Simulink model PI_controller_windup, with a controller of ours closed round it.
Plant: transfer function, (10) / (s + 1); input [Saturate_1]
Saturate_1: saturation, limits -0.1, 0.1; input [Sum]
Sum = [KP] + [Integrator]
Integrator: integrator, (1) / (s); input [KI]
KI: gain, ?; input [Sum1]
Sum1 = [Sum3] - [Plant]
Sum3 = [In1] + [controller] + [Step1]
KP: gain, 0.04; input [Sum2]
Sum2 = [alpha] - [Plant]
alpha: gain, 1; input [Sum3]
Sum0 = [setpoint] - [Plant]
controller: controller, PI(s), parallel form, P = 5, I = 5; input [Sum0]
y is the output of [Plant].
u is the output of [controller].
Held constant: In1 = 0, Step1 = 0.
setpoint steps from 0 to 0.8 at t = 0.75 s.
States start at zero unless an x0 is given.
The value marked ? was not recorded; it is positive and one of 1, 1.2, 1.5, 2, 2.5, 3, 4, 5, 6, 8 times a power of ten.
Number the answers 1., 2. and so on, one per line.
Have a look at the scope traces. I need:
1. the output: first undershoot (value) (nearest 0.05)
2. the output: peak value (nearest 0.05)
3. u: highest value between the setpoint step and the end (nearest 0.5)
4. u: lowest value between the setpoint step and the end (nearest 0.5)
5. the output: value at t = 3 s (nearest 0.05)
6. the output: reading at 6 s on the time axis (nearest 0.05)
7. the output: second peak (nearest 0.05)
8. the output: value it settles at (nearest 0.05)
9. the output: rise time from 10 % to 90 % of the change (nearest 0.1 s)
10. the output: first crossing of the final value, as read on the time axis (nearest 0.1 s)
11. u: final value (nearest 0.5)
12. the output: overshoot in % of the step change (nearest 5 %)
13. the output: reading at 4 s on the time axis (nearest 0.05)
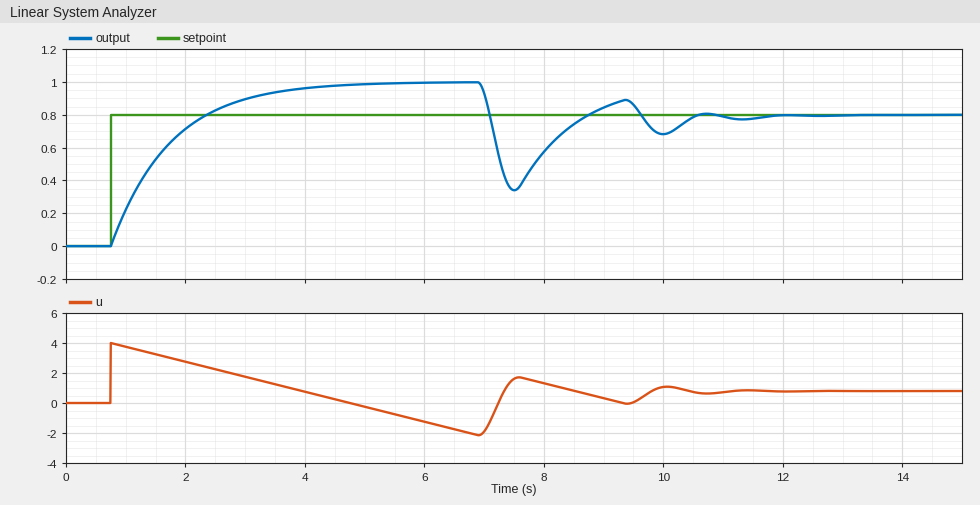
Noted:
1. 0.35
2. 1.00
3. 4.0
4. -2.0
5. 0.90
6. 1.00
7. 0.90
8. 0.80
9. 1.2 s
10. 2.4 s
11. 1.0
12. 25 %
13. 0.95
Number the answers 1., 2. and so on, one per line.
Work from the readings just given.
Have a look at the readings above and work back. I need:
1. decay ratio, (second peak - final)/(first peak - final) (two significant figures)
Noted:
1. 0.50
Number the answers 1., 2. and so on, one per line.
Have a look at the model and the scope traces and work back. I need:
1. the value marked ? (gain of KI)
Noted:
1. 0.4
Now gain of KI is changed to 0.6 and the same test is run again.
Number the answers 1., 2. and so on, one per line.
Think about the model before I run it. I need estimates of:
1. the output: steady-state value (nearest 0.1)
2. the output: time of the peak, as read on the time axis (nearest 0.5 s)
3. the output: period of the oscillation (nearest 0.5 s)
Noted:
1. 0.8
2. 7.0 s
3. 3.0 s
